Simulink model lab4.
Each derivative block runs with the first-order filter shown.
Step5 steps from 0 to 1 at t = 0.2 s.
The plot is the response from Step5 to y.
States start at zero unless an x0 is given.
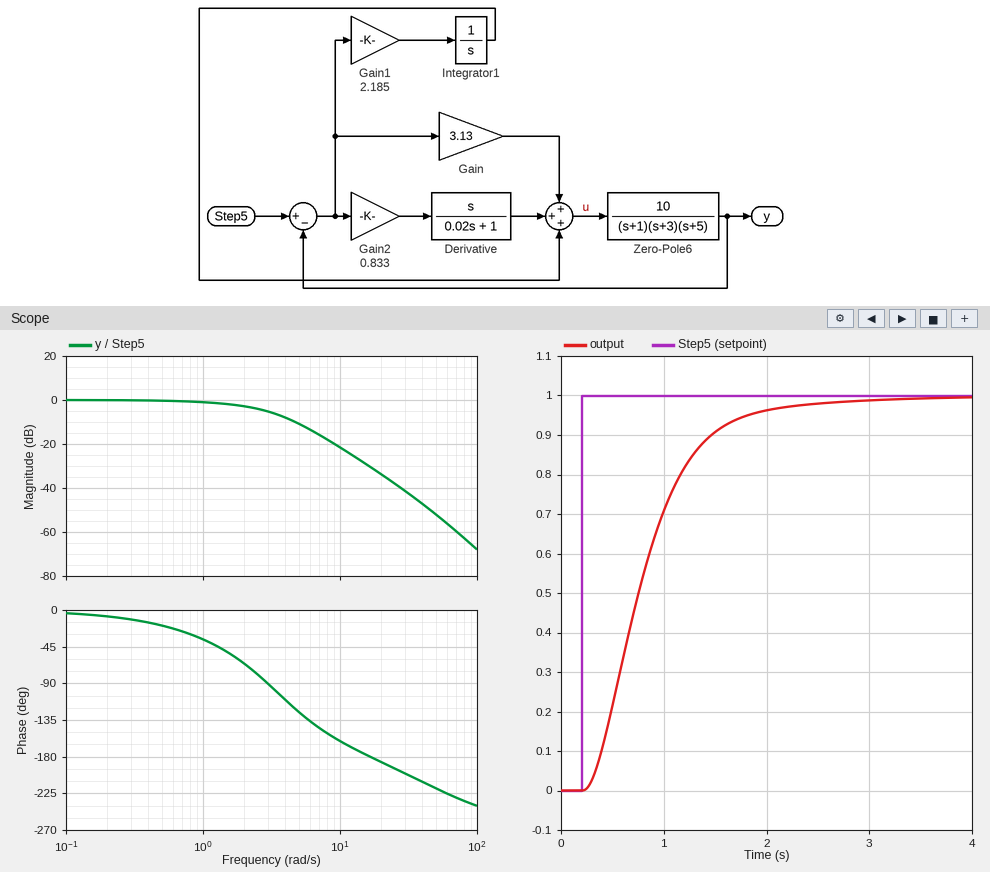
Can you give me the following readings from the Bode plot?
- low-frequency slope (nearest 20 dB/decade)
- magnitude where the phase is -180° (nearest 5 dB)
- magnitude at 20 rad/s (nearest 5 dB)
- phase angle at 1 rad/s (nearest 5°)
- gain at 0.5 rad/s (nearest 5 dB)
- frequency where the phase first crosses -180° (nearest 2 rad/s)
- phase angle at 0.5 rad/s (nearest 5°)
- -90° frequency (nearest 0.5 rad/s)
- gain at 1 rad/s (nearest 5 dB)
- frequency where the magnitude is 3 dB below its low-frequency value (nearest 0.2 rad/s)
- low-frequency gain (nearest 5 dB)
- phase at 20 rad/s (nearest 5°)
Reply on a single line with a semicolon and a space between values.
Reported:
0 dB/decade; -30 dB; -35 dB; -35°; 0 dB; 16 rad/s; -20°; 3.0 rad/s; 0 dB; 2.0 rad/s; 0 dB; -185°
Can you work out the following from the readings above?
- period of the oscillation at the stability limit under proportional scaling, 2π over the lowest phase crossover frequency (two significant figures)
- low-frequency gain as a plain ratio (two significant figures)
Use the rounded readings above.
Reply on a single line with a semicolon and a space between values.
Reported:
0.39 s; 1.0
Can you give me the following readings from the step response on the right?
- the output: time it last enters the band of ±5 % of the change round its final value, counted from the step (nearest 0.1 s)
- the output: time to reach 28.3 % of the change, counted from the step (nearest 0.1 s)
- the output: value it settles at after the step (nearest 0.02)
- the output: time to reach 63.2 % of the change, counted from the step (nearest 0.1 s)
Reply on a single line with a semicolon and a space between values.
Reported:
1.6 s; 0.4 s; 1.00; 0.7 s
